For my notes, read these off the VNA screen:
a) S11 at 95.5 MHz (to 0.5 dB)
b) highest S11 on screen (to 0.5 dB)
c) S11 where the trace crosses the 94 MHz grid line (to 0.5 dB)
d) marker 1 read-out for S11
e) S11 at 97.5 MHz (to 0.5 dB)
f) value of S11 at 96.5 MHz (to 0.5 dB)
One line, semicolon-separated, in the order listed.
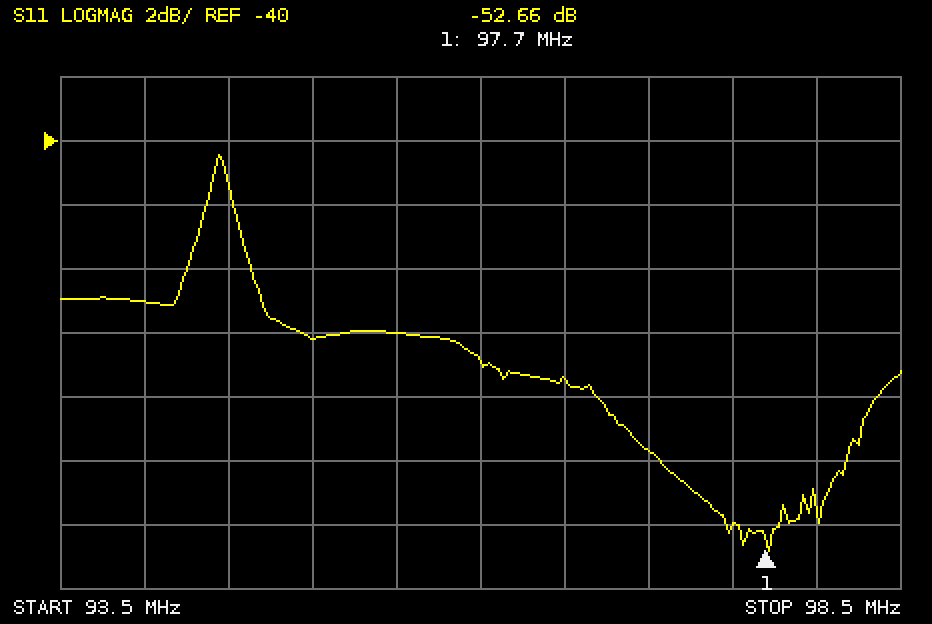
-46.0 dB; -40.5 dB; -45.0 dB; -52.66 dB; -52.0 dB; -47.5 dB
